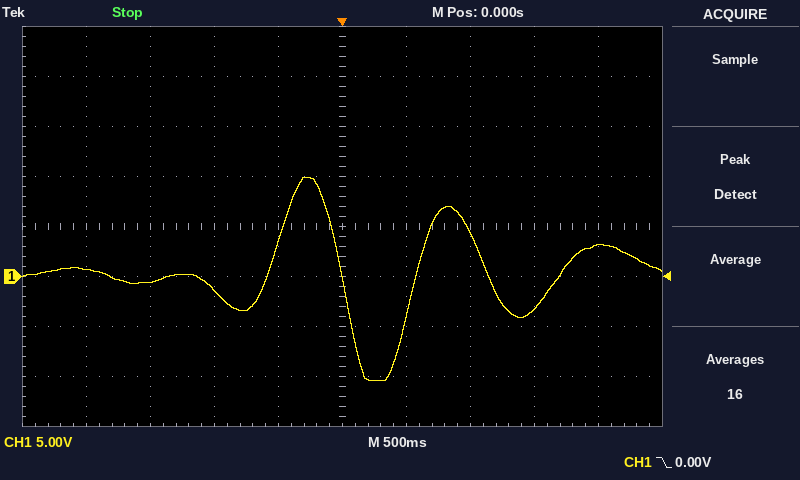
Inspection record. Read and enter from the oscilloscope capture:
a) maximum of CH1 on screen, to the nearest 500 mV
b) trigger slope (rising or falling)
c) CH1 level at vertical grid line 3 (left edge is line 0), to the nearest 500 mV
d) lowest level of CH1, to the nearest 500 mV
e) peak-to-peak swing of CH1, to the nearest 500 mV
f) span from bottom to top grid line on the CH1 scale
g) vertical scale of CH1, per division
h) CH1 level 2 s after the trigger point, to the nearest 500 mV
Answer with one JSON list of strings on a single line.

["10.0 V", "falling", "-1.5 V", "-10.5 V", "20.5 V", "40 V", "5 V", "3.0 V"]
